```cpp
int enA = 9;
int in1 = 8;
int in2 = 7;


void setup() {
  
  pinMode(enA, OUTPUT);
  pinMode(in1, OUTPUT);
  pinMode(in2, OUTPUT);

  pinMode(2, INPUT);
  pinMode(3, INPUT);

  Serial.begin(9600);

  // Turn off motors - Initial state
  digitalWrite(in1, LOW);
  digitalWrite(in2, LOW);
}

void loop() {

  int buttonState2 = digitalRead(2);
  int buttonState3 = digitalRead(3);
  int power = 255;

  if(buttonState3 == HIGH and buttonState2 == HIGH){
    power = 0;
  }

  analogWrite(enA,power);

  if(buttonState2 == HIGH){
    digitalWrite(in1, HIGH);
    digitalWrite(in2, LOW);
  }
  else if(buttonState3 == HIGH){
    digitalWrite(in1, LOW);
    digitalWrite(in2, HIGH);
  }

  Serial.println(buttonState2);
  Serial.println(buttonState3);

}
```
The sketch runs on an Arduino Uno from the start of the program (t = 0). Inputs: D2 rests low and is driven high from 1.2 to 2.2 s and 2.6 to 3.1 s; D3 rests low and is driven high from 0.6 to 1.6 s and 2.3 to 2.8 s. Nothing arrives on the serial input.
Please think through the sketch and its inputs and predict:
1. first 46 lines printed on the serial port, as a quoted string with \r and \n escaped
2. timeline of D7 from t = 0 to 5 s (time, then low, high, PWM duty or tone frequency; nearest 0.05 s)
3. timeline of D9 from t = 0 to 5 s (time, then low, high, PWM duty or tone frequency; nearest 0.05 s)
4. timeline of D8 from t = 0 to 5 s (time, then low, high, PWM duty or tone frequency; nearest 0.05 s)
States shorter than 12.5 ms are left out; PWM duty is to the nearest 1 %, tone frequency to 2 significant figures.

"0\r\n0\r\n0\r\n0\r\n0\r\n0\r\n0\r\n0\r\n0\r\n0\r\n0\r\n0\r\n0\r\n0\r\n0\r\n0\r\n0\r\n0\r\n0\r\n0\r\n0\r\n0\r\n0\r\n0\r\n0\r\n0\r\n0\r\n0\r\n0\r\n0\r\n0\r\n0\r\n0\r\n0\r\n0\r\n0\r\n0\r\n0\r\n0\r\n0\r\n0\r\n0\r\n0\r\n0\r\n0\r\n0\r\n"
0 s low; 0.6 s high; 1.2 s low; 2.3 s high; 2.6 s low
0 s high; 1.2 s low; 1.6 s high; 2.6 s low; 2.8 s high
0 s low; 1.2 s high; 2.3 s low; 2.6 s high
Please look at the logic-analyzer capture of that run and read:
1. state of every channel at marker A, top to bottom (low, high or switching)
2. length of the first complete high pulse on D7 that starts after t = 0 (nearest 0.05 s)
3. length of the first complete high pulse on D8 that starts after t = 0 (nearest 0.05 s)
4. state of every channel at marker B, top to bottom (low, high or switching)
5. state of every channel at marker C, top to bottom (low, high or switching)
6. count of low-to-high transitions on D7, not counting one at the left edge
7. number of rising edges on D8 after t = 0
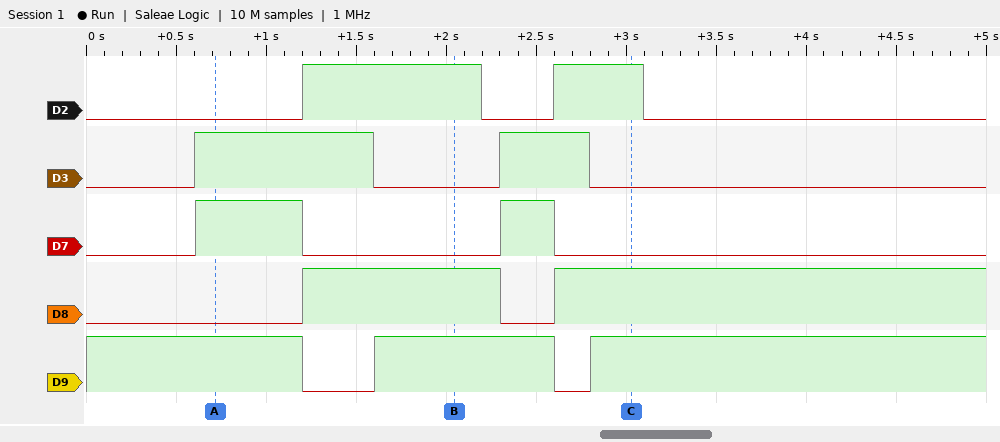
D2 low, D3 high, D7 high, D8 low, D9 high
0.60 s
1.10 s
D2 high, D3 low, D7 low, D8 high, D9 high
D2 high, D3 low, D7 low, D8 high, D9 high
2
2
